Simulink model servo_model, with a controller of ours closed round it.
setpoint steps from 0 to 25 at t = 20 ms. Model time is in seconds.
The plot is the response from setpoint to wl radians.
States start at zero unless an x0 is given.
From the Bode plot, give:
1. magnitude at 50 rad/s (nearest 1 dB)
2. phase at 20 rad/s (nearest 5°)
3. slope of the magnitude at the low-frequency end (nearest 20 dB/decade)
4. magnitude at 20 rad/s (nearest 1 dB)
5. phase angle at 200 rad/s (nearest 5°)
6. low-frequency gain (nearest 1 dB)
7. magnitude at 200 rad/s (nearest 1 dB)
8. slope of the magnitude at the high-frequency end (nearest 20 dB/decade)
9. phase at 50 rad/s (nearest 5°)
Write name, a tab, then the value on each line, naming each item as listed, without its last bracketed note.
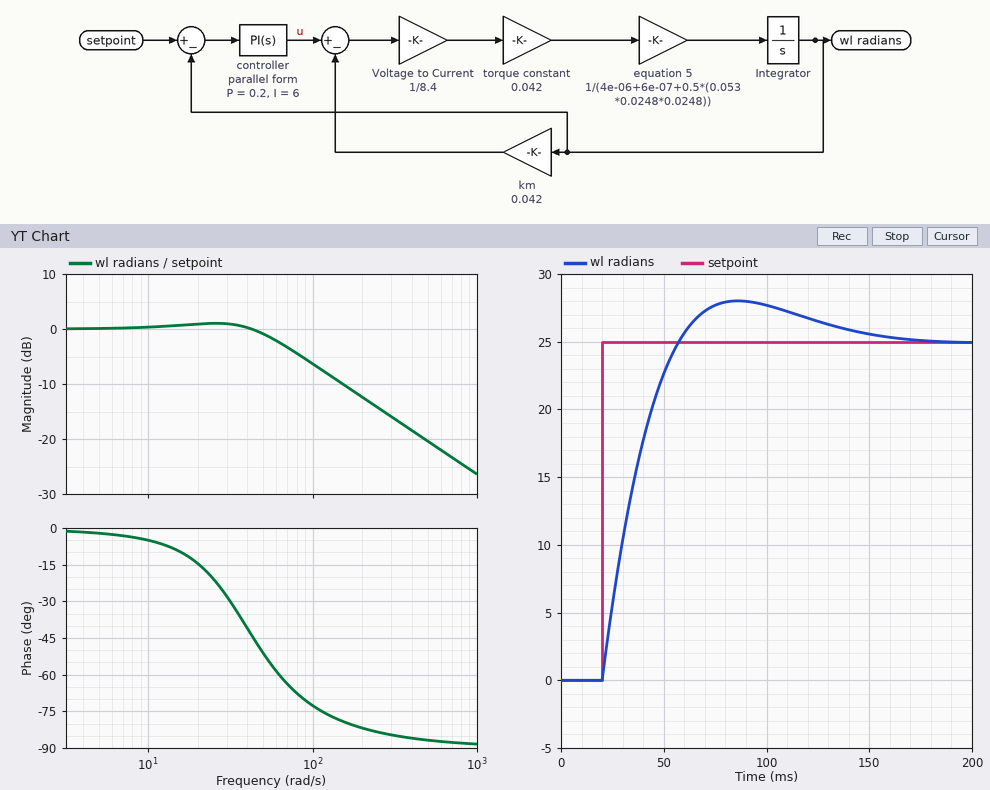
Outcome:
magnitude at 50 rad/s	-1 dB
phase at 20 rad/s	-15°
slope of the magnitude at the low-frequency end	0 dB/decade
magnitude at 20 rad/s	1 dB
phase angle at 200 rad/s	-80°
low-frequency gain	0 dB
magnitude at 200 rad/s	-12 dB
slope of the magnitude at the high-frequency end	-20 dB/decade
phase at 50 rad/s	-50°
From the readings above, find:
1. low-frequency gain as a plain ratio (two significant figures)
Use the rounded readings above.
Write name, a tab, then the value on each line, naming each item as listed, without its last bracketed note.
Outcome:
low-frequency gain as a plain ratio	1.0
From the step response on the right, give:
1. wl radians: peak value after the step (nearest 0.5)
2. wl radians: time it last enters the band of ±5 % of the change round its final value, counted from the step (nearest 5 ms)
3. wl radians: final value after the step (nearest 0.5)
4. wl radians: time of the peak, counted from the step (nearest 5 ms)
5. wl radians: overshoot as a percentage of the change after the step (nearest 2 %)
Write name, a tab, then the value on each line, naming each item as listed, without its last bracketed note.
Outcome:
wl radians: peak value after the step	28.0
wl radians: time it last enters the band of ±5 % of the change round its final value, counted from the step	110 ms
wl radians: final value after the step	25.0
wl radians: time of the peak, counted from the step	65 ms
wl radians: overshoot as a percentage of the change after the step	12 %
